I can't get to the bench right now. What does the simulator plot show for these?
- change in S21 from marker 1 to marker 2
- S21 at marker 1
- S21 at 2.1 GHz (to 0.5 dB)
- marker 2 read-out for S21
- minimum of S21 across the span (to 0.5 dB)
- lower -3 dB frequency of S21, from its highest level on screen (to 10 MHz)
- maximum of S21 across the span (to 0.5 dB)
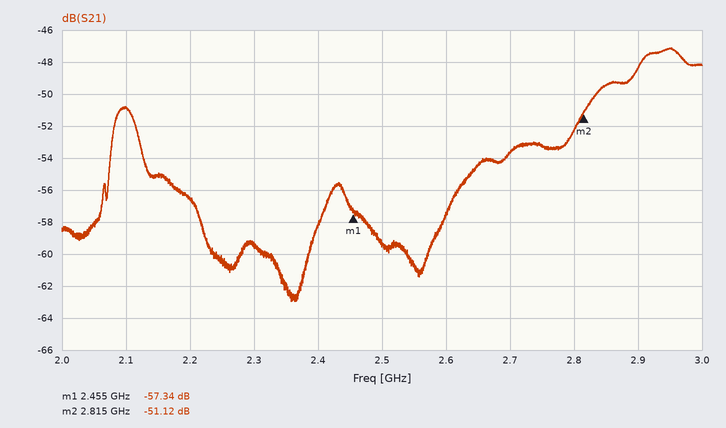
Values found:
6.22 dB
-57.34 dB
-51.0 dB
-51.12 dB
-63.0 dB
2.83 GHz
-47.0 dB
